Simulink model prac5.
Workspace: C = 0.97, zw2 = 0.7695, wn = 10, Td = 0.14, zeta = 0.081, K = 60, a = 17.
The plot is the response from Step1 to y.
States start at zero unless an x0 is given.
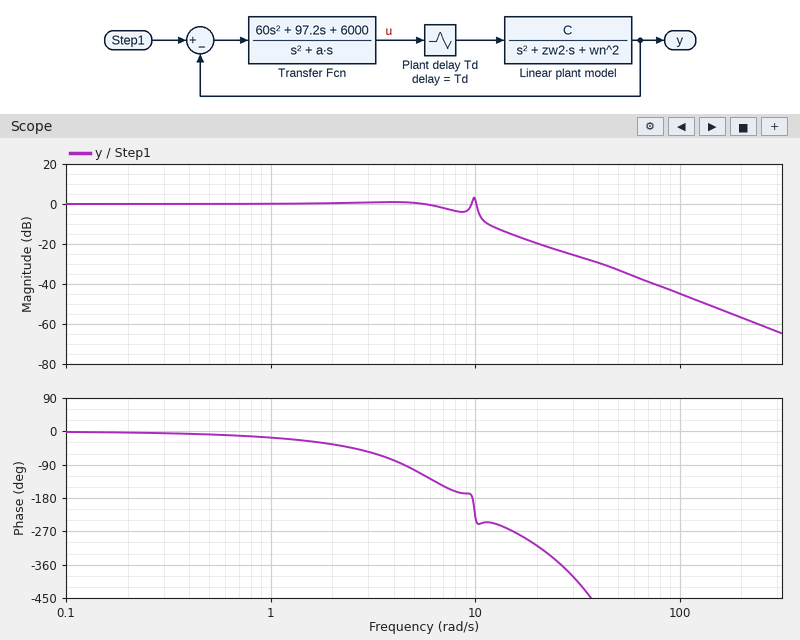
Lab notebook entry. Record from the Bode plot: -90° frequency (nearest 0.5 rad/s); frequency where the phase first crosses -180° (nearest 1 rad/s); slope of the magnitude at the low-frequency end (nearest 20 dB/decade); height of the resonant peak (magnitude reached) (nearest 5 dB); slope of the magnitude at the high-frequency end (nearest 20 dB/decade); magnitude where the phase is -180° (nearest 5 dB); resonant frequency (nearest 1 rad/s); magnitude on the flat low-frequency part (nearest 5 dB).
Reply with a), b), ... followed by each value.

a) 4.5 rad/s
b) 10 rad/s
c) 0 dB/decade
d) 5 dB
e) -40 dB/decade
f) 0 dB
g) 10 rad/s
h) 0 dB
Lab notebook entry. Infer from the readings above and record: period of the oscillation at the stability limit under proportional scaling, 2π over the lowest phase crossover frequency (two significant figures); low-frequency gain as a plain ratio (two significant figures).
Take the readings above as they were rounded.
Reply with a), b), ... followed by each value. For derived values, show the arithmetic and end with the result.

a) 2π / 10 = 0.63 s
b) 10^(0 / 20) = 1.0
